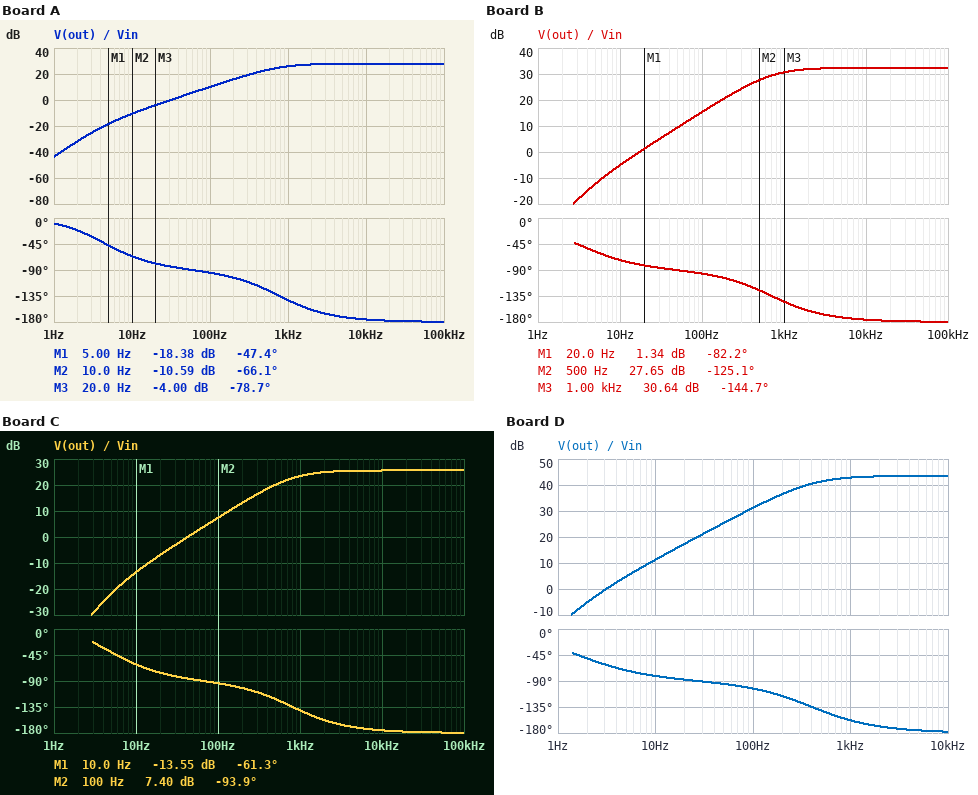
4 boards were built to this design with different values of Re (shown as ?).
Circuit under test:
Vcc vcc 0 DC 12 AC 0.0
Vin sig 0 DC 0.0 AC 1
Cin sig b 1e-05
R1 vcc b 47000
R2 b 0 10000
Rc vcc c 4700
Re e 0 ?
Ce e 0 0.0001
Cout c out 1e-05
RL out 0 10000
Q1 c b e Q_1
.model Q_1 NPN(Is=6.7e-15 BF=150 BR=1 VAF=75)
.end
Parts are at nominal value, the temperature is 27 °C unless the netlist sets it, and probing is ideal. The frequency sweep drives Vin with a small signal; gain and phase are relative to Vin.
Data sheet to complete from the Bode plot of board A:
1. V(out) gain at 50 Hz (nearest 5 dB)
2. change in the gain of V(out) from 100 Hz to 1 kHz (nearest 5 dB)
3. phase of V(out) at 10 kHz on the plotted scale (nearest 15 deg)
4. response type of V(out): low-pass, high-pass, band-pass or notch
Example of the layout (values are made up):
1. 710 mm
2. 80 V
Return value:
1. 5 dB
2. 15 dB
3. -180 deg
4. high-pass
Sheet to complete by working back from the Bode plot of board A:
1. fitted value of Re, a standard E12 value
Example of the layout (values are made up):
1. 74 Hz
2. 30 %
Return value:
1. 390 Ω
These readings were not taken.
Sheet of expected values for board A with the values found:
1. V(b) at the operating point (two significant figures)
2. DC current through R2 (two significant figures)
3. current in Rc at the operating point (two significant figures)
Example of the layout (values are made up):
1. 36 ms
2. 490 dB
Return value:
1. 1.6 V
2. 160 µA
3. 2.3 mA
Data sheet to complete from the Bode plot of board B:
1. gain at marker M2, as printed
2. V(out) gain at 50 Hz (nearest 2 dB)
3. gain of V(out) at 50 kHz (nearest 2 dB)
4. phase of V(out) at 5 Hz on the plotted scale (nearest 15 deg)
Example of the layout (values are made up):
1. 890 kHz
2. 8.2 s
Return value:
1. 27.65 dB
2. 10 dB
3. 32 dB
4. -60 deg
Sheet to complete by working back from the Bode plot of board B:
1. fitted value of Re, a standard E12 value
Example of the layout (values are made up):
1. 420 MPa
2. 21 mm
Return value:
1. 470 Ω
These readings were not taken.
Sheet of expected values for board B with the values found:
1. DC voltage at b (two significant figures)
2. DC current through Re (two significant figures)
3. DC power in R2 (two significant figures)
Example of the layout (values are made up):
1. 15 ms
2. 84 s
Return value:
1. 1.8 V
2. 2.3 mA
3. 320 µW
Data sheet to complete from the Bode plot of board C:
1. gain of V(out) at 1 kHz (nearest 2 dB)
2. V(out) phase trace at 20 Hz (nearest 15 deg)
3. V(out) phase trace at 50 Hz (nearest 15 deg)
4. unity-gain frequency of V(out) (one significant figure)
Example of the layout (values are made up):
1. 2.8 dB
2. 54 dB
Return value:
1. 24 dB
2. -75 deg
3. -90 deg
4. 40 Hz
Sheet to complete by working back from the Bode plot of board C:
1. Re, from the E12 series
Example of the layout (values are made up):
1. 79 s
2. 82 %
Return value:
1. 330 Ω
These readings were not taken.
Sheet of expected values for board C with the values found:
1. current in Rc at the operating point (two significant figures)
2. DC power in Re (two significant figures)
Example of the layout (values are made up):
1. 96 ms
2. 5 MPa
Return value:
1. 2.4 mA
2. 2.0 mW
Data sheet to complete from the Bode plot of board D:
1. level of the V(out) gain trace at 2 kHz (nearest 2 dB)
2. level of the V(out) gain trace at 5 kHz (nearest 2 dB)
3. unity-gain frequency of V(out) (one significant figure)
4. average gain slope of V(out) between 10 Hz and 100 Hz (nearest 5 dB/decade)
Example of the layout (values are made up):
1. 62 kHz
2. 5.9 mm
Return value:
1. 44 dB
2. 44 dB
3. 3 Hz
4. 20 dB/decade
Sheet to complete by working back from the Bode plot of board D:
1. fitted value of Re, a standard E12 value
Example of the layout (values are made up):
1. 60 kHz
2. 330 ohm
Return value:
1. 560 Ω
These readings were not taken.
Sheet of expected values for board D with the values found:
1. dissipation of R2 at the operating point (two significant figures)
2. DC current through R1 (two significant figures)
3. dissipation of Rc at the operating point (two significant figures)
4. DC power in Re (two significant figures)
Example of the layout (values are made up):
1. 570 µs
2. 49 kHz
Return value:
1. 380 µW
2. 210 µA
3. 24 mW
4. 2.9 mW
